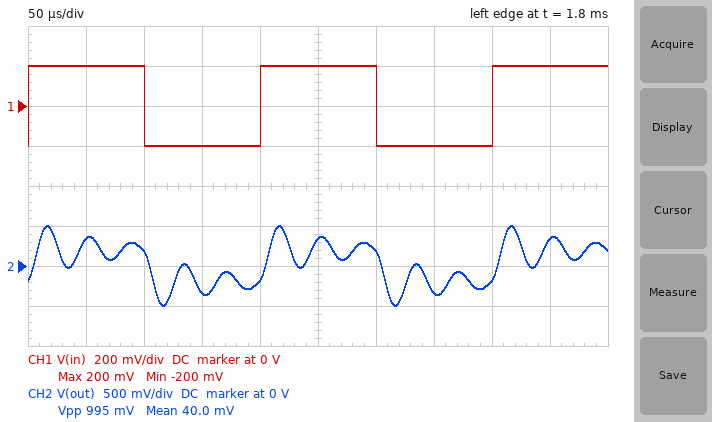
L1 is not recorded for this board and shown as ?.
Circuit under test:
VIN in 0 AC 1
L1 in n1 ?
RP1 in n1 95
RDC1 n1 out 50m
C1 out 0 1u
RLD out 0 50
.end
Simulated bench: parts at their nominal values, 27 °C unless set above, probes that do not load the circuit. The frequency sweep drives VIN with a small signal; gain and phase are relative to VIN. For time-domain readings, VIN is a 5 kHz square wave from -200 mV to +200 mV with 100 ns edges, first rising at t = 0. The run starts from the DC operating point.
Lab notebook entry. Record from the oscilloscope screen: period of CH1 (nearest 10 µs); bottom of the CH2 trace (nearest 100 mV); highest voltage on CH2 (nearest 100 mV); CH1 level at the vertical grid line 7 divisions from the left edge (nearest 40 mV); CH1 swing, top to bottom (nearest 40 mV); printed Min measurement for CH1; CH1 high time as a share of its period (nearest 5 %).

200 µs
-500 mV
500 mV
-200 mV
400 mV
-200 mV
50 %
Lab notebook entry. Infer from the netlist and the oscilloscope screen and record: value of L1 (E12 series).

33 µH
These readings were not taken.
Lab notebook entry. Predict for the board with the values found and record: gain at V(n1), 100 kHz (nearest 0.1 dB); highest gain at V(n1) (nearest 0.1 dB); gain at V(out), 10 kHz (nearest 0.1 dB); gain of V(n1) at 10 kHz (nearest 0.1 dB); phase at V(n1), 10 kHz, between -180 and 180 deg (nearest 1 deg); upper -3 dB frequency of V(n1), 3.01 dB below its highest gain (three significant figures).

-21.4 dB
14.8 dB
1.2 dB
1.2 dB
-3 deg
29.9 kHz
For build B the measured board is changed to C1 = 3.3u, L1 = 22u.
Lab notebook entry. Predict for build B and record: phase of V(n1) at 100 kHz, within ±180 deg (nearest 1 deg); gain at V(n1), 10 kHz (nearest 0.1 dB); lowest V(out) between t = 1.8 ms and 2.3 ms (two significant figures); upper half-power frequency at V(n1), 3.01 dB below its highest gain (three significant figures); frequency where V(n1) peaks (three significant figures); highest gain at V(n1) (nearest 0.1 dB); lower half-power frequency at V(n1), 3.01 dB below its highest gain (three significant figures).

-165 deg
2.9 dB
-440 mV
19.5 kHz
18.6 kHz
20.2 dB
17.7 kHz
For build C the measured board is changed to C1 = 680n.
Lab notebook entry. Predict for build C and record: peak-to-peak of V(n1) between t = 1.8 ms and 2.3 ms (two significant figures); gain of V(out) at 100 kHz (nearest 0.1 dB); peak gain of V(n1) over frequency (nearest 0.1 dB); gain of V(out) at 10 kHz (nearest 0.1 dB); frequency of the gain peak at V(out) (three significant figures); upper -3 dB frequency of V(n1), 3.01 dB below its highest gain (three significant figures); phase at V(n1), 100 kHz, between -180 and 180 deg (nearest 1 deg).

990 mV
-17.7 dB
13.2 dB
0.8 dB
33.2 kHz
36.7 kHz
-162 deg
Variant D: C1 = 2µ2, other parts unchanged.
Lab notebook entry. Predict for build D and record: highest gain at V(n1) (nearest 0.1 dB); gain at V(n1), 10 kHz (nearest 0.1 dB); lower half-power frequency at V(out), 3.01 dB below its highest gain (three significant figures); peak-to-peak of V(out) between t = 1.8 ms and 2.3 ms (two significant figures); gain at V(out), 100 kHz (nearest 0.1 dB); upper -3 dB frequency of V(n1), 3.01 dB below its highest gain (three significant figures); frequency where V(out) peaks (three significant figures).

17.7 dB
2.9 dB
17.3 kHz
890 mV
-28.6 dB
19.8 kHz
18.6 kHz
